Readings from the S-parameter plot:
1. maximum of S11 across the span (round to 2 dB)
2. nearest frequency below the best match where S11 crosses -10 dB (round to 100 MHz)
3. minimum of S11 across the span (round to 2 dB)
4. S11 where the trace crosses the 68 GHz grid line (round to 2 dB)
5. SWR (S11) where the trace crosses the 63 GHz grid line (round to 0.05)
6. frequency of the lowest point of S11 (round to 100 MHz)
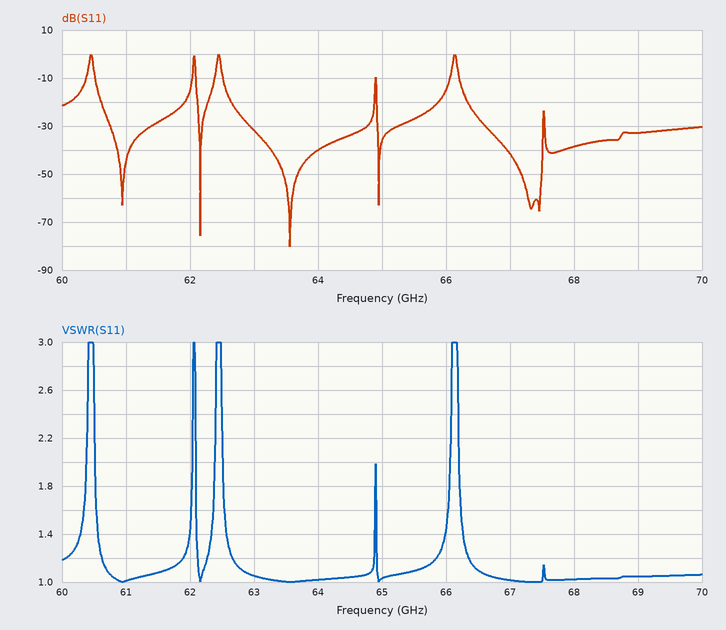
0 dB
62.5 GHz
-80 dB
-38 dB
1.05
63.6 GHz
